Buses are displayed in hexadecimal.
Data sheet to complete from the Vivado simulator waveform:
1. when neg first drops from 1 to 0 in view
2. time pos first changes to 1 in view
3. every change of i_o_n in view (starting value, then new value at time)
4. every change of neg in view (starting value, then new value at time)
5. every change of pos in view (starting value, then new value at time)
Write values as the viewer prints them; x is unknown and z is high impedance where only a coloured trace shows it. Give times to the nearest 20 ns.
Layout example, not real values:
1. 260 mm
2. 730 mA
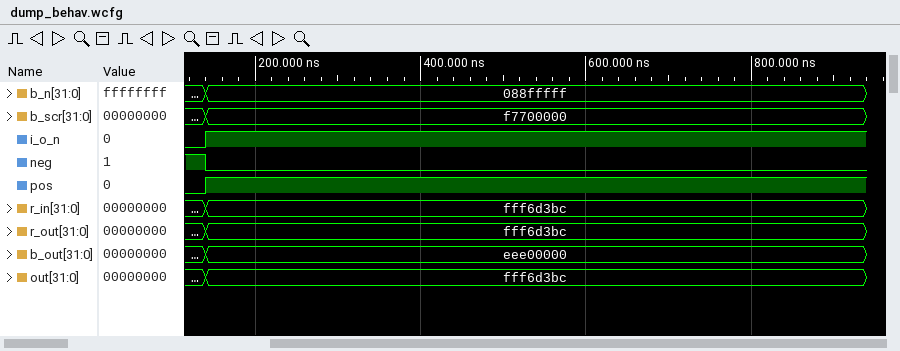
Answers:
1. 140 ns
2. 140 ns
3. 0, 1 at 140 ns
4. 1, 0 at 140 ns
5. 0, 1 at 140 ns
